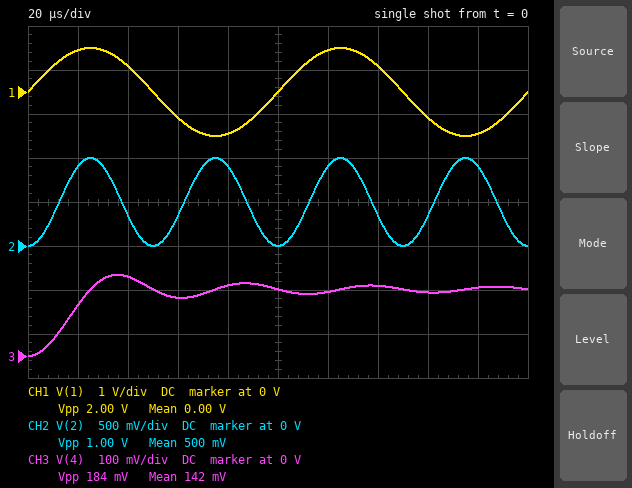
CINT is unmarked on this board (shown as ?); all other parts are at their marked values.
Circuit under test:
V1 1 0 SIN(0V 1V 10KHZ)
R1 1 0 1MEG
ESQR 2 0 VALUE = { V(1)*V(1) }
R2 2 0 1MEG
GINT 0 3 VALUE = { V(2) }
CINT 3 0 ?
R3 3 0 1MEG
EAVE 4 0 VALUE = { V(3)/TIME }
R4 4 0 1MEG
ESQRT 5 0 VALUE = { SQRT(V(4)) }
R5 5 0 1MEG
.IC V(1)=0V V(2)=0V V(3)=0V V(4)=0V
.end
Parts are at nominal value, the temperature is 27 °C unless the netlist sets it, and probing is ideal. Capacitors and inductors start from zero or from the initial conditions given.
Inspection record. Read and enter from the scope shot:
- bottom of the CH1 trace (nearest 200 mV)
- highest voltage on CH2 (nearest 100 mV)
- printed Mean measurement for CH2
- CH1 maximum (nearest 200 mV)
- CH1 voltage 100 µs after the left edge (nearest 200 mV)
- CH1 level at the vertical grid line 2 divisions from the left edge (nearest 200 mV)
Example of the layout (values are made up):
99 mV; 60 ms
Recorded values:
-1.0 V; 1.0 V; 500 mV; 1.0 V; 0 V; 600 mV
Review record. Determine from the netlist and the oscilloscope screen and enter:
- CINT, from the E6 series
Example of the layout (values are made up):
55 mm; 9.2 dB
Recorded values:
3.3 F
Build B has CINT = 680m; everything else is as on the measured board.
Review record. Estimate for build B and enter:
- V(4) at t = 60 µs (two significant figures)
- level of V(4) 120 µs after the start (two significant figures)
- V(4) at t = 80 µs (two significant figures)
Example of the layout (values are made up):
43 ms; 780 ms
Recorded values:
640 mV; 710 mV; 780 mV
